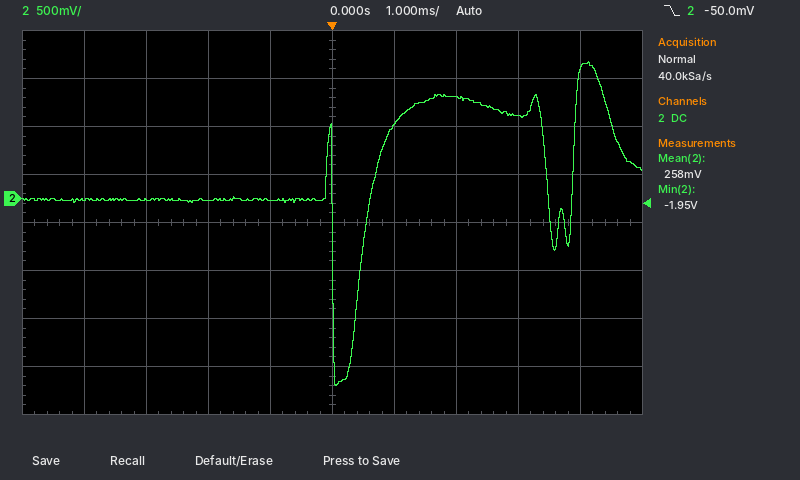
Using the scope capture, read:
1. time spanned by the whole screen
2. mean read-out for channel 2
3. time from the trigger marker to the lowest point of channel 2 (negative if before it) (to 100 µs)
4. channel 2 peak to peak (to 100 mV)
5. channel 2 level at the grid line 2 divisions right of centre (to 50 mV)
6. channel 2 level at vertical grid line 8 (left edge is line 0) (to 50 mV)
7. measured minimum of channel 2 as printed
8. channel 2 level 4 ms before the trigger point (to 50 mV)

10 ms
258 mV
+100 µs
3.40 V
1.05 V
850 mV
-1.95 V
0 mV
